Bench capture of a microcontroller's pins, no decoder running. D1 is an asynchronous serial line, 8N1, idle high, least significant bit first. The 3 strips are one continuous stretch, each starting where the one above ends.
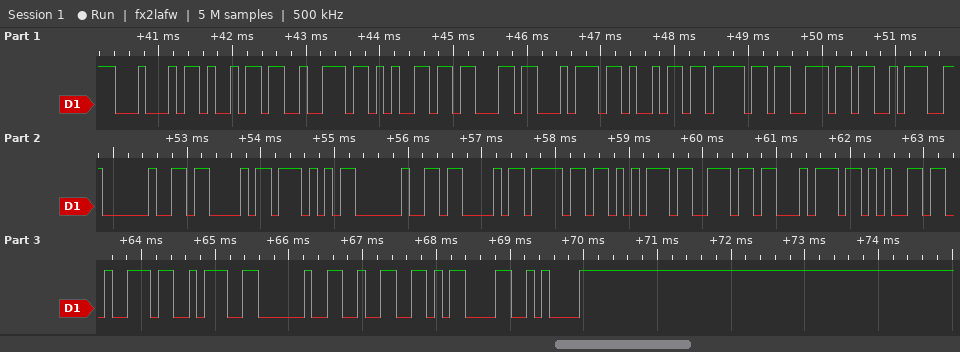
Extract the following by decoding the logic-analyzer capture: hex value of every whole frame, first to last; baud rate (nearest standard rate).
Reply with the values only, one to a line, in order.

44 69 72 65 63 74 69 6F 6E 3A 20 43 57 20 43 6F 75 6E 74 65 72 3A 20 32 0D 0A
9600 baud
